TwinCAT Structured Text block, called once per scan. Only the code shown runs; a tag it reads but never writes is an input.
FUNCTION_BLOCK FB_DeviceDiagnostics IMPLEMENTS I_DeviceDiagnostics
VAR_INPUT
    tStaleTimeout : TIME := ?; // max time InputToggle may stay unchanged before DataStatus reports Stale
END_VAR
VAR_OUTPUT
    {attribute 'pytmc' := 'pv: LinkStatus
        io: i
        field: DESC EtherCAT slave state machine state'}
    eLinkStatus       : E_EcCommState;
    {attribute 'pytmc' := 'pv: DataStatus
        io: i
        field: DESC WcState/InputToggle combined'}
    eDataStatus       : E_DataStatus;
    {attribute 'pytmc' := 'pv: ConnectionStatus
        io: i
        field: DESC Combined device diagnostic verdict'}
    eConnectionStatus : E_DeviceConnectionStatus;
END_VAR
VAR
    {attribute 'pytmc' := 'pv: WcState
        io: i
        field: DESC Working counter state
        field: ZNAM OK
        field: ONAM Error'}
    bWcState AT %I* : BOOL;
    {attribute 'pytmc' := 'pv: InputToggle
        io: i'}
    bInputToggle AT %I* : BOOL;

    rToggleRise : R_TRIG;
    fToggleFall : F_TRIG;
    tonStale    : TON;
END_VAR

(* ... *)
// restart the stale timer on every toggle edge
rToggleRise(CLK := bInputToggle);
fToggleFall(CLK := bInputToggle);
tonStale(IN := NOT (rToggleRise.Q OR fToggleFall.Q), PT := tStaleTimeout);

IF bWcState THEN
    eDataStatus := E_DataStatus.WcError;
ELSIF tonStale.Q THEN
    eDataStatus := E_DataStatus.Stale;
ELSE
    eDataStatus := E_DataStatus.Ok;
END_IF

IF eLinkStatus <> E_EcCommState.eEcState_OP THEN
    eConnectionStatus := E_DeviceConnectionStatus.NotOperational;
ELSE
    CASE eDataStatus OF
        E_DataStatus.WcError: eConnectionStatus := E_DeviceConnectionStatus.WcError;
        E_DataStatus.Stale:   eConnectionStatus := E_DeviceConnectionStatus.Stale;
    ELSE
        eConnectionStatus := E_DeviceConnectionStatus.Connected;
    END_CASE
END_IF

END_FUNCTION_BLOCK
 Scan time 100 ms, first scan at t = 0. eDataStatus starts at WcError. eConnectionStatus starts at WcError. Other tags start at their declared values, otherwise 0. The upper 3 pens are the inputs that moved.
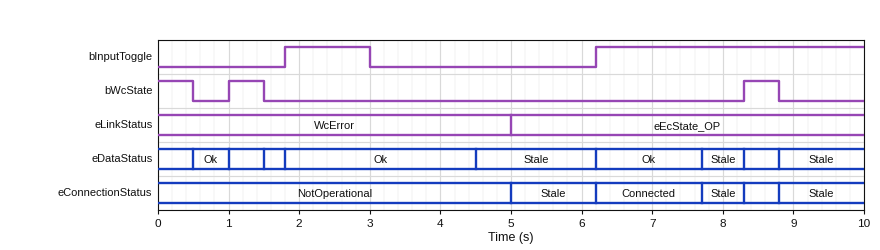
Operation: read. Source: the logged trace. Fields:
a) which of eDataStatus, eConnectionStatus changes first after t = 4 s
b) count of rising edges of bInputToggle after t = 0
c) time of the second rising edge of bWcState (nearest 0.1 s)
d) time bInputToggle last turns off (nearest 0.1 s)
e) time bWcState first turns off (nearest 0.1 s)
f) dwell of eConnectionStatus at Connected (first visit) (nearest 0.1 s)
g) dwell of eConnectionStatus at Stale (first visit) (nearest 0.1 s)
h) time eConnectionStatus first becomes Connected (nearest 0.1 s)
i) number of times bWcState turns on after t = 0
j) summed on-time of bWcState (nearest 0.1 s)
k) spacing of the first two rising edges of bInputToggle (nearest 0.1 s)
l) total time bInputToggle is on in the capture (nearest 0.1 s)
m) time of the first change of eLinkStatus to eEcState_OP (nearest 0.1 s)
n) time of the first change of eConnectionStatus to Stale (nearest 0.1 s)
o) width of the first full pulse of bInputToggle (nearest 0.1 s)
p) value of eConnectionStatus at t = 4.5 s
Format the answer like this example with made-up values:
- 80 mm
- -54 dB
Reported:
- eDataStatus
- 2
- 8.3 s
- 3.0 s
- 0.5 s
- 1.5 s
- 1.2 s
- 6.2 s
- 2
- 1.5 s
- 4.4 s
- 5.0 s
- 5.0 s
- 5.0 s
- 1.2 s
- NotOperational
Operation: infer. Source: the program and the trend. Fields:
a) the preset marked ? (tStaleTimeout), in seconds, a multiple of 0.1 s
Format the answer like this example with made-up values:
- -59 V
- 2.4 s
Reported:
- 1.4 s
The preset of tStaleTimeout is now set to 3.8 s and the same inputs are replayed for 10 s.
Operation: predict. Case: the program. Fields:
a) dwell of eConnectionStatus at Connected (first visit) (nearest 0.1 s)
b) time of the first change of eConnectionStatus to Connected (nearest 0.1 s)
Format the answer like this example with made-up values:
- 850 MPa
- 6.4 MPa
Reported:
- 3.3 s
- 5.0 s
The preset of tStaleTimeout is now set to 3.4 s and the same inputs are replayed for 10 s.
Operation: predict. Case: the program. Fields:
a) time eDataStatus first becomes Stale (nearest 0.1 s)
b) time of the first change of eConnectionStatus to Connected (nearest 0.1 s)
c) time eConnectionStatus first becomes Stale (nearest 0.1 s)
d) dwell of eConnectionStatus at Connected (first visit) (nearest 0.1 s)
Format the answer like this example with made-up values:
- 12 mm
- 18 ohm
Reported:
- 9.7 s
- 5.0 s
- 9.7 s
- 3.3 s
